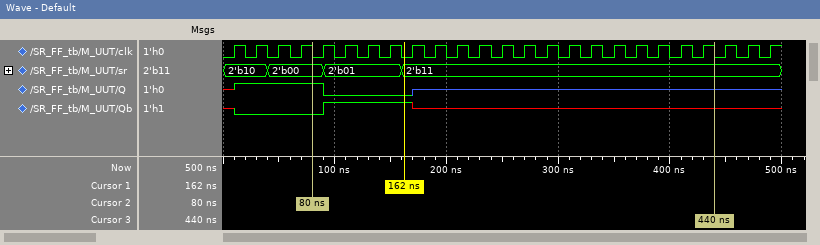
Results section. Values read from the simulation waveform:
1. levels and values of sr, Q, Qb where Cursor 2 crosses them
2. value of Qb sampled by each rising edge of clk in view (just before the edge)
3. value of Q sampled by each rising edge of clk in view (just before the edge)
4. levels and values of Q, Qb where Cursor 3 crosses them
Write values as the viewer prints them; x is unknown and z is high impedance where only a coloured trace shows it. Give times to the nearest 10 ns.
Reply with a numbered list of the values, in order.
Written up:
1. sr=2'b00, Q=1, Qb=0
2. x 0 0 0 0 1 1 1 1 x x x x x x x x x x x x x x x x
3. x 1 1 1 1 0 0 0 0 z z z z z z z z z z z z z z z z
4. Q=z, Qb=x
